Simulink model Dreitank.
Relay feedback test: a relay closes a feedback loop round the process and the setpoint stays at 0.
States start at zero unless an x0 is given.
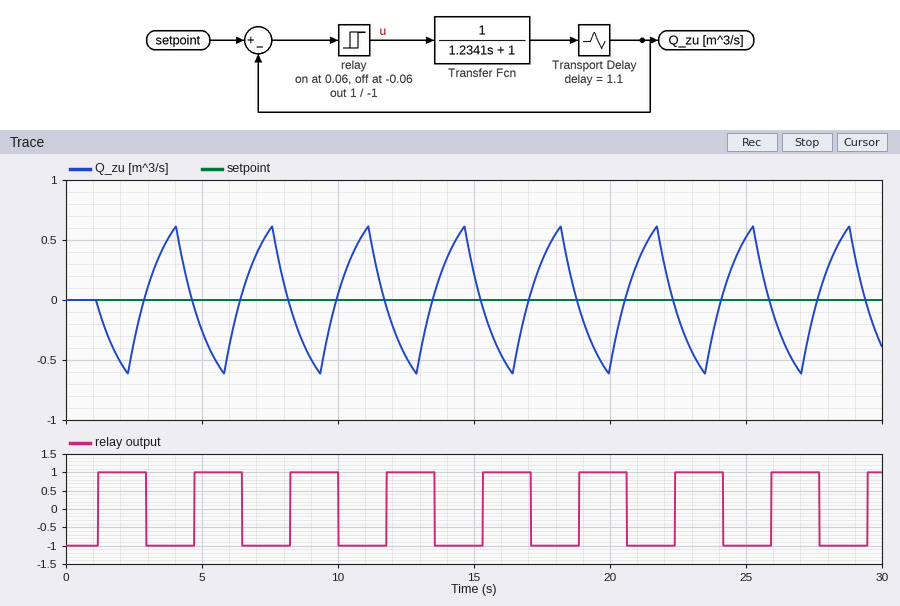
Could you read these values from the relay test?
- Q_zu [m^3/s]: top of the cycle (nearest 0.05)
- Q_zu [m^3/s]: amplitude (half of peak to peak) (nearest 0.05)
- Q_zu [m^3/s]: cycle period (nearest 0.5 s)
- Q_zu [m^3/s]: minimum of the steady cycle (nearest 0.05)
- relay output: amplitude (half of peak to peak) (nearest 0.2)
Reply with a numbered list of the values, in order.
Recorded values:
1. 0.60
2. 0.60
3. 3.5 s
4. -0.60
5. 1.0
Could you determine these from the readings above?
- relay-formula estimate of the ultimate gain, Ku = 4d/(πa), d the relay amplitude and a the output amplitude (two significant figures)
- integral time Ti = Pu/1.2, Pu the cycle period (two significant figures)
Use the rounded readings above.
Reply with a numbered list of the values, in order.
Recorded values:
1. 2.1
2. 2.9 s
